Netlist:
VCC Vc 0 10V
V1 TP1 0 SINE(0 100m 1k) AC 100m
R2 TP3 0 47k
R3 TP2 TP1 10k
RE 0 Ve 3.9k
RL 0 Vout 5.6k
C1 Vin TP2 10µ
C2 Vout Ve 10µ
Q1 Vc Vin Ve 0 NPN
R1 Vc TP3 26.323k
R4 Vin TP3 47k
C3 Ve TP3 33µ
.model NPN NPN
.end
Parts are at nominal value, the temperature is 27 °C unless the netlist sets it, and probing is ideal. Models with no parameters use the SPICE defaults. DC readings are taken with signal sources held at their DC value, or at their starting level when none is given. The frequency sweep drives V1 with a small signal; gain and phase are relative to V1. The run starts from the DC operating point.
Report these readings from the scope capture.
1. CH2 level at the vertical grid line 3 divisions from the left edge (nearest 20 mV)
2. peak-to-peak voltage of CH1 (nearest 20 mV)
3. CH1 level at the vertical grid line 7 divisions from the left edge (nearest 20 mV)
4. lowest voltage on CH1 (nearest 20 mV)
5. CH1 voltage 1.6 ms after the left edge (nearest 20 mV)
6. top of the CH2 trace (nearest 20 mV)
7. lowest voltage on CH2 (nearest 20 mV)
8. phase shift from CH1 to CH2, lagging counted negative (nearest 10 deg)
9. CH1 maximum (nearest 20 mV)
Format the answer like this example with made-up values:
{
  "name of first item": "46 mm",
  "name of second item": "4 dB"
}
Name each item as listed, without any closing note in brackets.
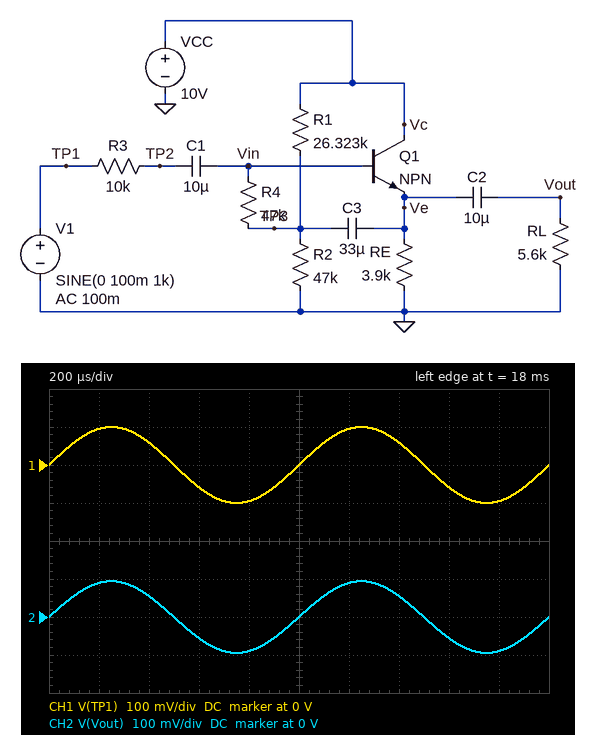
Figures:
{
  "CH2 level at the vertical grid line 3 divisions from the left edge": "-60 mV",
  "peak-to-peak voltage of CH1": "200 mV",
  "CH1 level at the vertical grid line 7 divisions from the left edge": "60 mV",
  "lowest voltage on CH1": "-100 mV",
  "CH1 voltage 1.6 ms after the left edge": "-60 mV",
  "top of the CH2 trace": "100 mV",
  "lowest voltage on CH2": "-100 mV",
  "phase shift from CH1 to CH2, lagging counted negative": "0 deg",
  "CH1 maximum": "100 mV"
}
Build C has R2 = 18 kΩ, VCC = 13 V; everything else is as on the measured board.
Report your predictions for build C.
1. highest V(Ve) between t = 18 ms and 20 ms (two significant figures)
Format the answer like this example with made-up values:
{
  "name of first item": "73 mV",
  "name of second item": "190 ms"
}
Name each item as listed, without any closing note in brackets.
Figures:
{
  "highest V(Ve) between t = 18 ms and 20 ms": "4.0 V"
}
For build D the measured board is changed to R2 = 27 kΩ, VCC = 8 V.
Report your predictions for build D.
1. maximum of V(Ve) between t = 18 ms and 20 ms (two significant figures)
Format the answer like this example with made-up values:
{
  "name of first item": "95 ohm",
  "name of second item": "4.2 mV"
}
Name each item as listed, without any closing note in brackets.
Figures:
{
  "maximum of V(Ve) between t = 18 ms and 20 ms": "2.9 V"
}
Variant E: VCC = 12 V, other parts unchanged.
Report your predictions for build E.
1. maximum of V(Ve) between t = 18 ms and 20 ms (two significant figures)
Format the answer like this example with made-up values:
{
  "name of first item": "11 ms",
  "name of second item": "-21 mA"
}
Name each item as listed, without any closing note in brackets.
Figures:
{
  "maximum of V(Ve) between t = 18 ms and 20 ms": "6.0 V"
}
